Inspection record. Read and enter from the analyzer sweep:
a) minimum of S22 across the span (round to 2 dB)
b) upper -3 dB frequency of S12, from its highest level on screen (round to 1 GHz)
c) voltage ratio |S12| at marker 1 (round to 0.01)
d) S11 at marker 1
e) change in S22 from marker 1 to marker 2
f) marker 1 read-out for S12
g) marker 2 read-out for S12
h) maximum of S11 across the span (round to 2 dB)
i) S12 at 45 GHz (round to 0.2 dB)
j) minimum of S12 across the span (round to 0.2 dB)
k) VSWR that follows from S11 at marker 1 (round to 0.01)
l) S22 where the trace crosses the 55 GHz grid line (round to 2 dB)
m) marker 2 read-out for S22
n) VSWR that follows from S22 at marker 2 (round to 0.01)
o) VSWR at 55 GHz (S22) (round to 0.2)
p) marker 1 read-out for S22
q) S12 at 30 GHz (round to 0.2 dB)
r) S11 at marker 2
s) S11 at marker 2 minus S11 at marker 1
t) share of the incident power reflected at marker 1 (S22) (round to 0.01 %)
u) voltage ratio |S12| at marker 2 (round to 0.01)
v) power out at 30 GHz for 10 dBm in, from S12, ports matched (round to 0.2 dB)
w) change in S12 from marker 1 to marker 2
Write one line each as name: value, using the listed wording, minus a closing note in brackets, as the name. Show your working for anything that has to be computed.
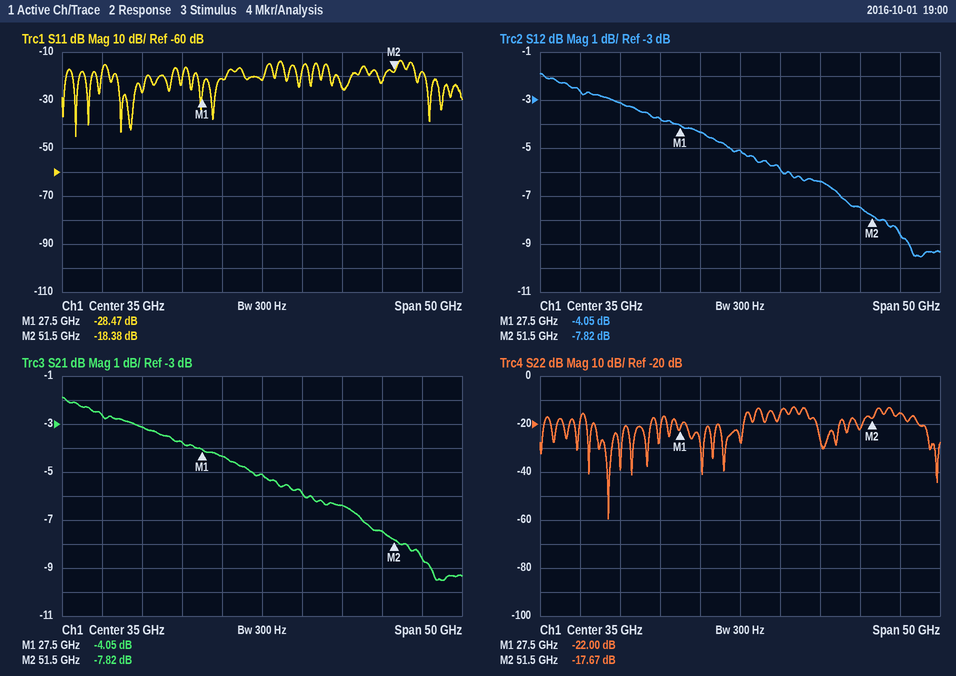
minimum of S22 across the span: -60 dB
upper -3 dB frequency of S12, from its highest level on screen: 33 GHz
voltage ratio |S12| at marker 1: 10^(-4.05/20) ≈ 0.63
S11 at marker 1: -28.47 dB
change in S22 from marker 1 to marker 2: -17.67 − (-22) = 4.33 dB
marker 1 read-out for S12: -4.05 dB
marker 2 read-out for S12: -7.82 dB
maximum of S11 across the span: -14 dB
S12 at 45 GHz: -6.4 dB
minimum of S12 across the span: -9.6 dB
VSWR that follows from S11 at marker 1: (1 + 0.0377)/(1 − 0.0377) ≈ 1.08
S22 where the trace crosses the 55 GHz grid line: -16 dB
marker 2 read-out for S22: -17.67 dB
VSWR that follows from S22 at marker 2: (1 + 0.1308)/(1 − 0.1308) ≈ 1.30
VSWR at 55 GHz (S22): |Γ| = 10^(-16/20) = 0.1585; VSWR = (1 + 0.1585)/(1 − 0.1585) ≈ 1.4
marker 1 read-out for S22: -22.00 dB
S12 at 30 GHz: -4.4 dB
S11 at marker 2: -18.38 dB
S11 at marker 2 minus S11 at marker 1: -18.38 − (-28.47) = 10.09 dB
share of the incident power reflected at marker 1 (S22): 10^(-22/10) ≈ 0.63 %
voltage ratio |S12| at marker 2: 10^(-7.82/20) ≈ 0.41
power out at 30 GHz for 10 dBm in, from S12, ports matched: 10 dBm + (-4.4 dB) = 5.6 dBm
change in S12 from marker 1 to marker 2: -7.82 − (-4.05) = -3.77 dB
